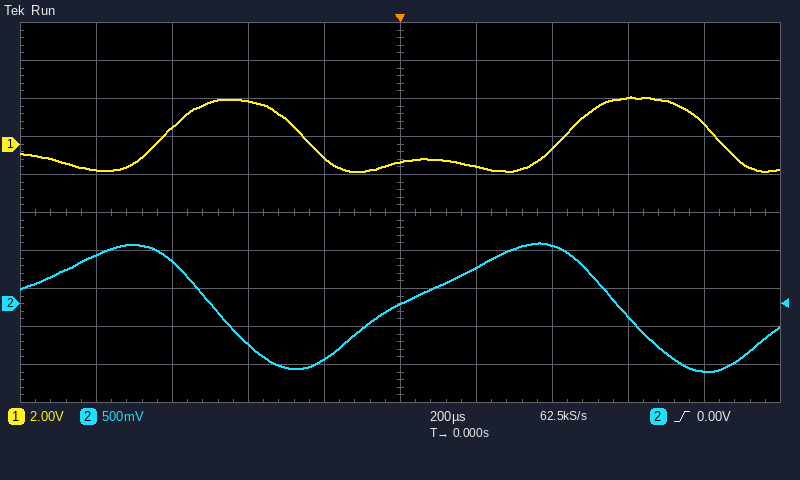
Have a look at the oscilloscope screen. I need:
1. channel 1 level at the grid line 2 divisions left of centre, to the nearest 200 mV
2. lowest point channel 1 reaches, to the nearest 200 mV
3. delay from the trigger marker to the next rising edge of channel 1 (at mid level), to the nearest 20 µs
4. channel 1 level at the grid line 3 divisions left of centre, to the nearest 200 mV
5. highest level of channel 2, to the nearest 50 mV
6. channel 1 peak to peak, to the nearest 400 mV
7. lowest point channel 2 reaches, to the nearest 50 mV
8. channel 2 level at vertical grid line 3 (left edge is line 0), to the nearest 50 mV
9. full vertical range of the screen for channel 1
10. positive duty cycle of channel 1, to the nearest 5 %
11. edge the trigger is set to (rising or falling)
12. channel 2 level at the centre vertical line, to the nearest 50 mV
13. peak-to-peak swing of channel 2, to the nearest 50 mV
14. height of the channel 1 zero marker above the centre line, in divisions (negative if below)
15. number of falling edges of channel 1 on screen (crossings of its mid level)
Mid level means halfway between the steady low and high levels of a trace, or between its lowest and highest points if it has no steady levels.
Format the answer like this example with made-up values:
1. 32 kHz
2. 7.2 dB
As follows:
1. 2.2 V
2. -1.4 V
3. 440 µs
4. 800 mV
5. 800 mV
6. 4.0 V
7. -900 mV
8. -550 mV
9. 20 V
10. 35 %
11. rising
12. 0 mV
13. 1.70 V
14. +1.8 div
15. 2
